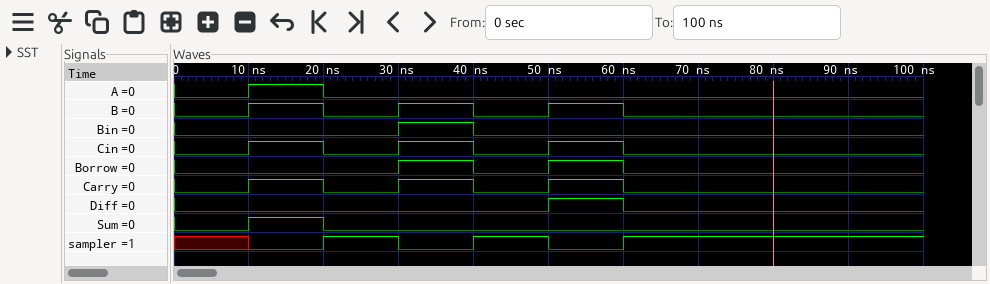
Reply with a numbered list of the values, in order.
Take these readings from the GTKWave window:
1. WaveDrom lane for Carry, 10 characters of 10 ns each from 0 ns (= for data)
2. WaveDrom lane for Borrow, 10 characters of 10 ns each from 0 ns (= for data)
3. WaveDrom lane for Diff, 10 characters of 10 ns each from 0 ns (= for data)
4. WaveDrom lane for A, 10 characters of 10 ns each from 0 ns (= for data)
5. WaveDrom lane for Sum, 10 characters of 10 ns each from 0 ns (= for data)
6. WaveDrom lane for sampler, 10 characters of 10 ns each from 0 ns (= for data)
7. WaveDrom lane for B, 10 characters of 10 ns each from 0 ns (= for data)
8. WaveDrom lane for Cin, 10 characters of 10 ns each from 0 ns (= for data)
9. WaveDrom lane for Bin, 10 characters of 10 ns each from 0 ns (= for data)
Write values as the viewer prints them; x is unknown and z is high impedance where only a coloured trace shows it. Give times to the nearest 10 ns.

1. {name: 'Carry', wave: '0101010...'}
2. {name: 'Borrow', wave: '0..1010...'}
3. {name: 'Diff', wave: '0....10...'}
4. {name: 'A', wave: '010.......'}
5. {name: 'Sum', wave: '010.......'}
6. {name: 'sampler', wave: 'x010101...'}
7. {name: 'B', wave: '0101010...'}
8. {name: 'Cin', wave: '0101010...'}
9. {name: 'Bin', wave: '0..10.....'}
